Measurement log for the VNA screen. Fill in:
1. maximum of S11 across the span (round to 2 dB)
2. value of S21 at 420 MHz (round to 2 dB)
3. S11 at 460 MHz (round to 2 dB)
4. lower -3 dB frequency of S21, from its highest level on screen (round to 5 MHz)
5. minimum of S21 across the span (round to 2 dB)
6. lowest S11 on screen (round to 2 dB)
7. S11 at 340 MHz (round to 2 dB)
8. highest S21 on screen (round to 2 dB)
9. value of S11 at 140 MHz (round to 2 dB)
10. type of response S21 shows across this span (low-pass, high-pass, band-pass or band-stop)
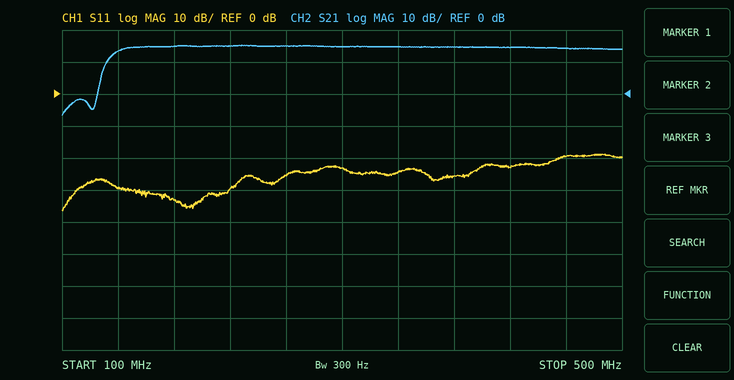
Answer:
-18 dB
14 dB
-20 dB
135 MHz
-6 dB
-36 dB
-24 dB
16 dB
-30 dB
high-pass
